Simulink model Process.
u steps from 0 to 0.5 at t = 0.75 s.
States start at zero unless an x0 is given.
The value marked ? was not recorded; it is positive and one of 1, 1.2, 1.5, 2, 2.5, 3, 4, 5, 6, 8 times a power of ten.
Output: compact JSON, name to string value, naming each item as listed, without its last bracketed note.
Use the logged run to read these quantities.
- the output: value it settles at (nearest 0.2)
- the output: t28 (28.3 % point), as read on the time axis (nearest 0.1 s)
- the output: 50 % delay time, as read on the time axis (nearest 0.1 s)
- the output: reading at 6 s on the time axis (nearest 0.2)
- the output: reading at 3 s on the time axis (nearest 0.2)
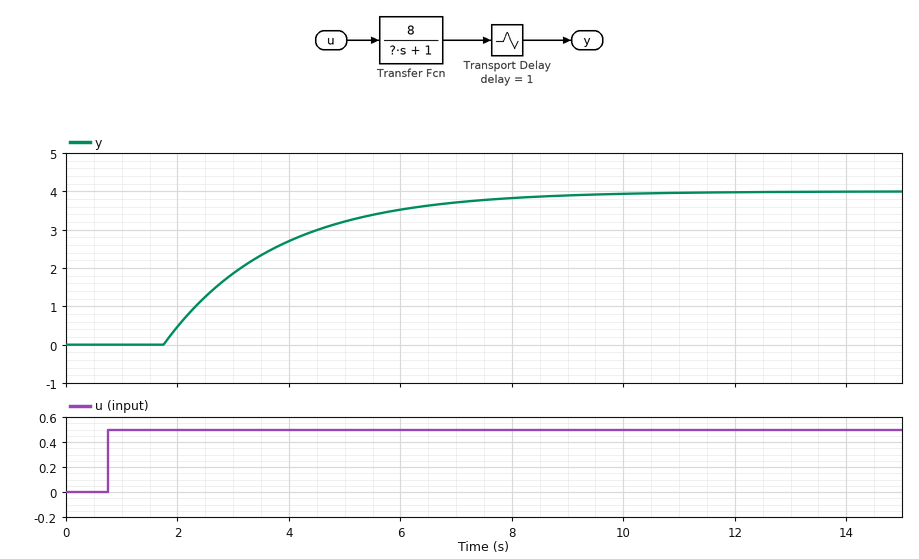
{"the output: value it settles at": "4.0", "the output: t28 (28.3 % point), as read on the time axis": "2.4 s", "the output: 50 % delay time, as read on the time axis": "3.1 s", "the output: reading at 6 s on the time axis": "3.6", "the output: reading at 3 s on the time axis": "1.8"}
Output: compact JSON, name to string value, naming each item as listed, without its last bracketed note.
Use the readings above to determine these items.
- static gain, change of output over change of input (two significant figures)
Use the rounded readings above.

{"static gain, change of output over change of input": "8.0"}
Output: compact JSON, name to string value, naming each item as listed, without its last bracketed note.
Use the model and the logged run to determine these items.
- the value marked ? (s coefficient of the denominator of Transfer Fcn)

{"the value marked ?": "2"}
